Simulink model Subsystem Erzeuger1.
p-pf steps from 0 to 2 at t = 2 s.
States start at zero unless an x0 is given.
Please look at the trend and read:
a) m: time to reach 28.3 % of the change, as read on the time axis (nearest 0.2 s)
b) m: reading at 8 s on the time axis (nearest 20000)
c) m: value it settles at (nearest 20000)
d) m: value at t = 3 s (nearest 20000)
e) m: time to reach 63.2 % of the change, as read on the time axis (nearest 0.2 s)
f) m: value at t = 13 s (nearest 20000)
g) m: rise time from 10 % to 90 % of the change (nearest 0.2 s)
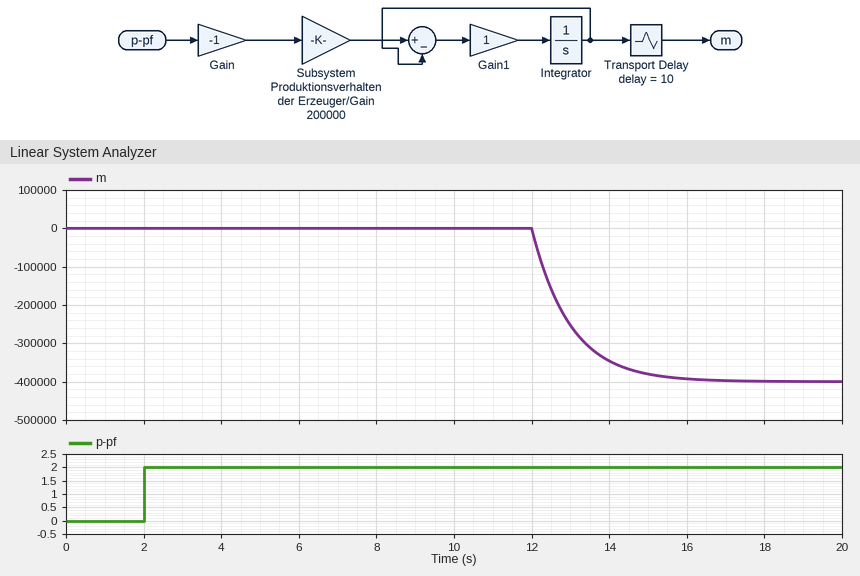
12.4 s
0
-400000
0
13.0 s
-260000
2.2 s
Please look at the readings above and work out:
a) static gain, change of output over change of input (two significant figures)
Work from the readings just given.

-200000
